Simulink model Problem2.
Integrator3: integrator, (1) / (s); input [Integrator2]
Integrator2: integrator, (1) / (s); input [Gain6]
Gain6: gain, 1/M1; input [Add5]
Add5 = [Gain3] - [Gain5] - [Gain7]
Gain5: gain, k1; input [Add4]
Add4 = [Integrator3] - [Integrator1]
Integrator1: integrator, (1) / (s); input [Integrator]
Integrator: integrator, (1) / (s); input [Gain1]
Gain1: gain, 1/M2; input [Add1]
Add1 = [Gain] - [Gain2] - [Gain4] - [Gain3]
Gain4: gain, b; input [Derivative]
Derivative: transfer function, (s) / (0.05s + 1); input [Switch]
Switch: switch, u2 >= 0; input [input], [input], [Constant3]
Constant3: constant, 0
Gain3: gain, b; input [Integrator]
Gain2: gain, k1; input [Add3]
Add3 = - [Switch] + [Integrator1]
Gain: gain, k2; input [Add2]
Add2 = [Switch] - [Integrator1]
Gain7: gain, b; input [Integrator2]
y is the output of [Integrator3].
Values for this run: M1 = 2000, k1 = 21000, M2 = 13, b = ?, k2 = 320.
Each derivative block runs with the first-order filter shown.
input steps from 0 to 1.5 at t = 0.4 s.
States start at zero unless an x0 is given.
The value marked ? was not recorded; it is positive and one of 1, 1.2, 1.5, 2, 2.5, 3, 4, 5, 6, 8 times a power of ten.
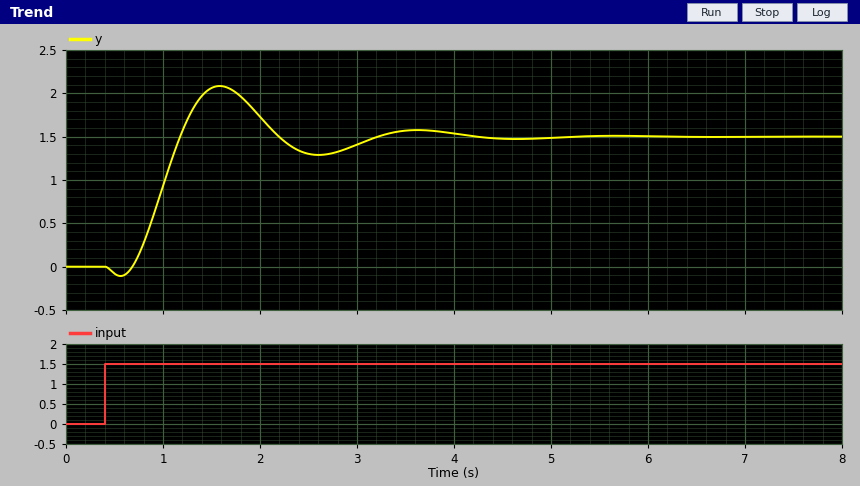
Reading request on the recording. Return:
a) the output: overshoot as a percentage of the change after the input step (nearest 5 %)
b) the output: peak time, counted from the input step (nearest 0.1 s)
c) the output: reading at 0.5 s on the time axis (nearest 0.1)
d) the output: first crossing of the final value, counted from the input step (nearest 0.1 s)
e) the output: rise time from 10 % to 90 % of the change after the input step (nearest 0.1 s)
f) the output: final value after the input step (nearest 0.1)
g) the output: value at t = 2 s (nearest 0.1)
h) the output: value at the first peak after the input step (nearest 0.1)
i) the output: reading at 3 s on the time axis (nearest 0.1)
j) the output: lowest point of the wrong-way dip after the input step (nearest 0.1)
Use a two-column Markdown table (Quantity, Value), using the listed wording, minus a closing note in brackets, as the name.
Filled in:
| Quantity | Value |
|---|---|
| the output: overshoot as a percentage of the change after the input step | 40 % |
| the output: peak time, counted from the input step | 1.2 s |
| the output: reading at 0.5 s on the time axis | -0.1 |
| the output: first crossing of the final value, counted from the input step | 0.8 s |
| the output: rise time from 10 % to 90 % of the change after the input step | 0.4 s |
| the output: final value after the input step | 1.5 |
| the output: value at t = 2 s | 1.7 |
| the output: value at the first peak after the input step | 2.1 |
| the output: reading at 3 s on the time axis | 1.4 |
| the output: lowest point of the wrong-way dip after the input step | -0.1 |
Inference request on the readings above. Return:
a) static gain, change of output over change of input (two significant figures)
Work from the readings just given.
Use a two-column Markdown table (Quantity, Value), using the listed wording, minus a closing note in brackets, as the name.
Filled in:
| Quantity | Value |
|---|---|
| static gain, change of output over change of input | 1.0 |
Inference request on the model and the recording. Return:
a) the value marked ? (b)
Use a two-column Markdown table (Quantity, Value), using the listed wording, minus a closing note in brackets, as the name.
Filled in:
| Quantity | Value |
|---|---|
| the value marked ? | 4000 |
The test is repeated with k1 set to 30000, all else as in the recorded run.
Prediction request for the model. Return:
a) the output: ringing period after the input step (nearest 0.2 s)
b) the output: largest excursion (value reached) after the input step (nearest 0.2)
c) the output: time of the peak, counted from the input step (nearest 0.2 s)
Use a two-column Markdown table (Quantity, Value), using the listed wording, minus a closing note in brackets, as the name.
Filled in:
| Quantity | Value |
|---|---|
| the output: ringing period after the input step | 1.6 s |
| the output: largest excursion (value reached) after the input step | 2.2 |
| the output: time of the peak, counted from the input step | 1.0 s |
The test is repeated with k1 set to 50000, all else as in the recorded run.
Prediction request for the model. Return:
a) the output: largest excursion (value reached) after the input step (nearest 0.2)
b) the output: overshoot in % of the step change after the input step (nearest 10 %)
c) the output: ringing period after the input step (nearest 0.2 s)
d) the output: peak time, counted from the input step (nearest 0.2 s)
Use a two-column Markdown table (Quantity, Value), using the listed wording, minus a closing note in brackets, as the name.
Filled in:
| Quantity | Value |
|---|---|
| the output: largest excursion (value reached) after the input step | 2.2 |
| the output: overshoot in % of the step change after the input step | 50 % |
| the output: ringing period after the input step | 1.2 s |
| the output: peak time, counted from the input step | 0.8 s |
